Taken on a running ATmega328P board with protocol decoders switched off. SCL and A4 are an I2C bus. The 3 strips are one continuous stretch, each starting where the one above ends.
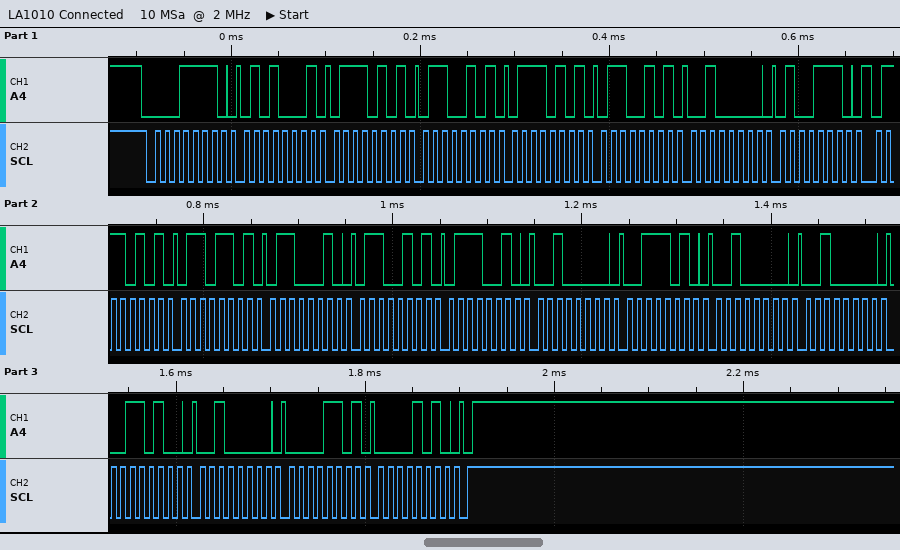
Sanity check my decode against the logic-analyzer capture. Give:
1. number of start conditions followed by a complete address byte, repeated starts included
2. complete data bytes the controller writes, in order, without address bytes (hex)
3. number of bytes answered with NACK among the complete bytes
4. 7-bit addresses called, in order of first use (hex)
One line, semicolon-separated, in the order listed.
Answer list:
1; 51 75 65 75 65 20 4E 75 6D 62 65 72 20 3A 20 20 34 20 0D 0A; 0; 0x0F
